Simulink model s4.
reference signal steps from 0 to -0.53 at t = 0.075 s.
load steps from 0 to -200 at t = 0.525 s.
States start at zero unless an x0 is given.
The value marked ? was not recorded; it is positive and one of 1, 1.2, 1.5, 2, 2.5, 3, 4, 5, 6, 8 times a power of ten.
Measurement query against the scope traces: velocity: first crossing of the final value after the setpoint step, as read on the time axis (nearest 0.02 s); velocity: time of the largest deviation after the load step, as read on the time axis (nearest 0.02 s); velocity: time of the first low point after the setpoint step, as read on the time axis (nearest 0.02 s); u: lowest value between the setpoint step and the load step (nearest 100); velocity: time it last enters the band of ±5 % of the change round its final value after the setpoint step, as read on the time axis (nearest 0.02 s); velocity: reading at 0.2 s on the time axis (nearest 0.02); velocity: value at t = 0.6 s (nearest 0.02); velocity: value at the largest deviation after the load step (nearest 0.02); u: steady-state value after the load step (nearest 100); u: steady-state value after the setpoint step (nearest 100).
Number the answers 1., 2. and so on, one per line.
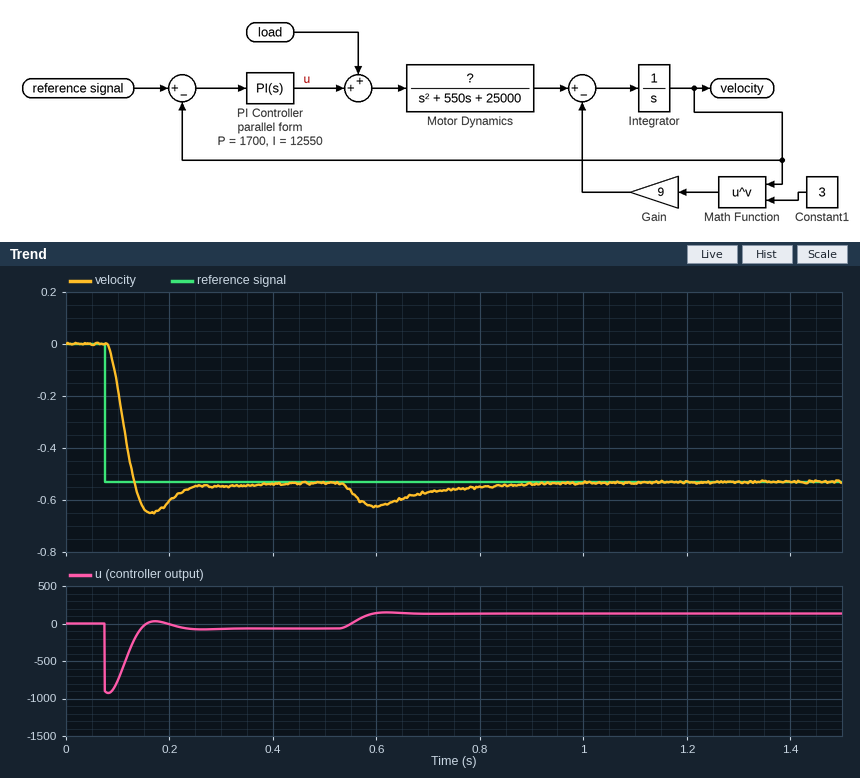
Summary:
1. 0.14 s
2. 0.60 s
3. 0.16 s
4. -900
5. 0.24 s
6. -0.60
7. -0.62
8. -0.62
9. 100
10. -100
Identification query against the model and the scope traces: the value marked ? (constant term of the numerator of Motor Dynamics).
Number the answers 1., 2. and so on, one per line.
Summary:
1. 500
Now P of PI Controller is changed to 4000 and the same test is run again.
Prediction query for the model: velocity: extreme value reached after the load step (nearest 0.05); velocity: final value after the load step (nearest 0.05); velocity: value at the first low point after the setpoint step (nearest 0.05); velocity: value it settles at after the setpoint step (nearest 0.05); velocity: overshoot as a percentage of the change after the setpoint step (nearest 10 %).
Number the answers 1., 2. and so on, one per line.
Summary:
1. -0.60
2. -0.55
3. -0.70
4. -0.55
5. 30 %
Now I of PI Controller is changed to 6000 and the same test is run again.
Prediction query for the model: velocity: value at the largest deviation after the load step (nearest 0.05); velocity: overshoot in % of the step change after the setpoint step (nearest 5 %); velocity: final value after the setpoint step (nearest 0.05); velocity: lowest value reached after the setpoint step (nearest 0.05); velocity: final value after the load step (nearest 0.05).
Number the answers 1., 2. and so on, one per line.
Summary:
1. -0.65
2. 15 %
3. -0.55
4. -0.60
5. -0.55
